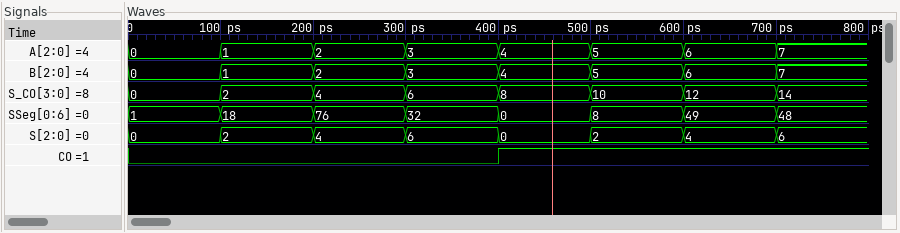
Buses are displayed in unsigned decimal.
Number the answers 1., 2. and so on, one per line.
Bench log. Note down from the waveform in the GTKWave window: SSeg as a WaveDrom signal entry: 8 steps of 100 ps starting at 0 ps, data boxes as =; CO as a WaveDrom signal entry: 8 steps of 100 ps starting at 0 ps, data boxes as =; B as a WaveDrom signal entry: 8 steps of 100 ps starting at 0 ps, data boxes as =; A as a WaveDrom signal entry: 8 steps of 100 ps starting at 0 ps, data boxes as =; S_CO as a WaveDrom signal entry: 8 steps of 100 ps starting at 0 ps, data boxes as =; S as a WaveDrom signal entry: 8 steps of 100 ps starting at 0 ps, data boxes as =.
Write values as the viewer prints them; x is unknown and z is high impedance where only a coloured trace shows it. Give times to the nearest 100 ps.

1. {name: 'SSeg', wave: '========', data: '1 18 76 32 0 8 49 48'}
2. {name: 'CO', wave: '0...1...'}
3. {name: 'B', wave: '========', data: '0 1 2 3 4 5 6 7'}
4. {name: 'A', wave: '========', data: '0 1 2 3 4 5 6 7'}
5. {name: 'S_CO', wave: '========', data: '0 2 4 6 8 10 12 14'}
6. {name: 'S', wave: '========', data: '0 2 4 6 0 2 4 6'}
